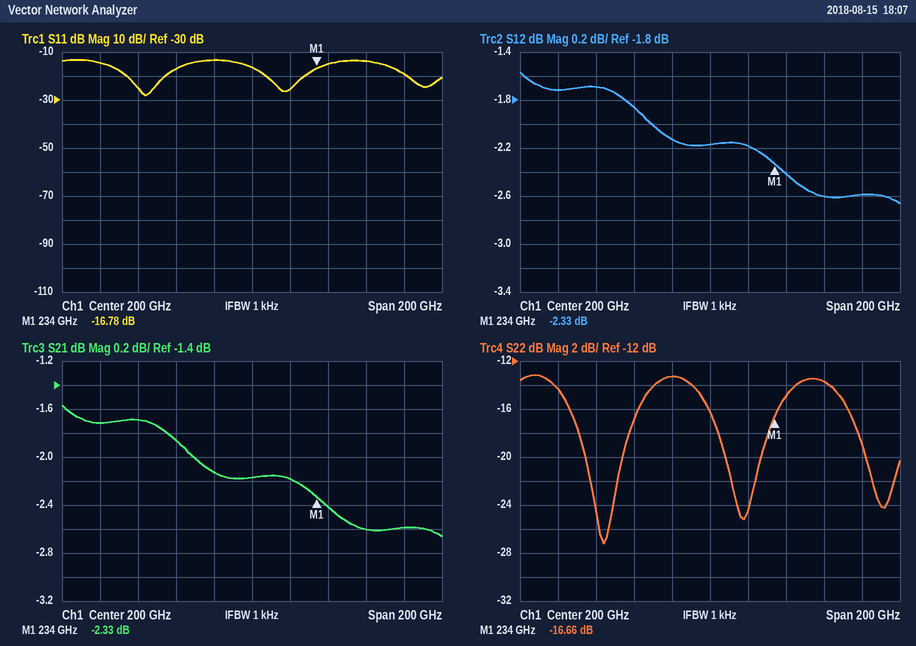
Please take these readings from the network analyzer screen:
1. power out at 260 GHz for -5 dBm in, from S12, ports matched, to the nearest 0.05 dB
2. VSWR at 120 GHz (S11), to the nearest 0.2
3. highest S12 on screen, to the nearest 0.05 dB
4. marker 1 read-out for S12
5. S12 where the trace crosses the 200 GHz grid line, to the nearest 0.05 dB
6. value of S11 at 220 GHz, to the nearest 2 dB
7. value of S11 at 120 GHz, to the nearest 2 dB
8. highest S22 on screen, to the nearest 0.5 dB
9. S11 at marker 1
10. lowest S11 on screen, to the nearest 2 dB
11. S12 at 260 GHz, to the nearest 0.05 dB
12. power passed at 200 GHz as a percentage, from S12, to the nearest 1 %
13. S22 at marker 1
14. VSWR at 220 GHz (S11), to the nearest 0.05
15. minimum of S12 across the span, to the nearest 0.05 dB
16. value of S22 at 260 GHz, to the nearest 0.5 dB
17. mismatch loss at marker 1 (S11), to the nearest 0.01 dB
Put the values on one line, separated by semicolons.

-7.60 dBm; 1.4; -1.55 dB; -2.33 dB; -2.15 dB; -26 dB; -14 dB; -13.0 dB; -16.78 dB; -28 dB; -2.60 dB; 61 %; -16.66 dB; 1.10; -2.65 dB; -13.5 dB; 0.09 dB
